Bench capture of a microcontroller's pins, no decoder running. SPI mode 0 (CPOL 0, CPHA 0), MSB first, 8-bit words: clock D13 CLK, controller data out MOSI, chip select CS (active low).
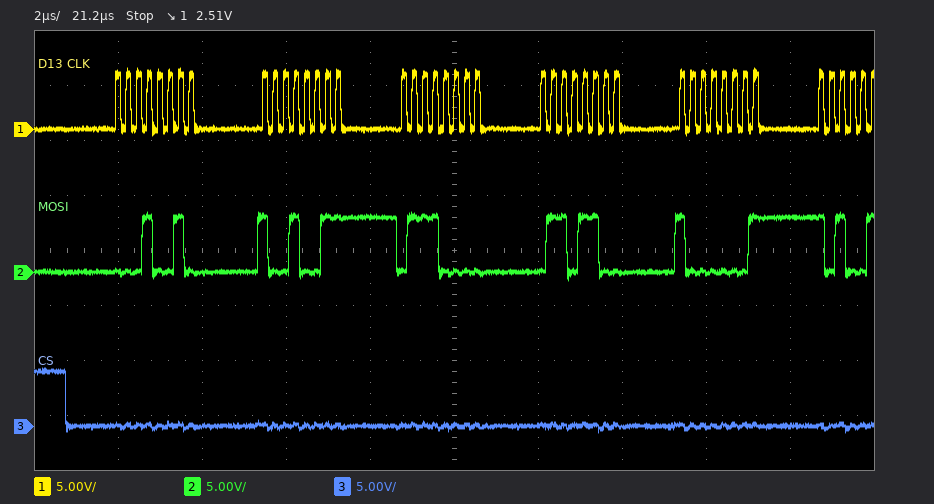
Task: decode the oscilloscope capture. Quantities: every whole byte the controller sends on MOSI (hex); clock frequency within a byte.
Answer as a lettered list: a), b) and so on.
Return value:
a) 12 93 70 6C 81
b) 4 MHz
